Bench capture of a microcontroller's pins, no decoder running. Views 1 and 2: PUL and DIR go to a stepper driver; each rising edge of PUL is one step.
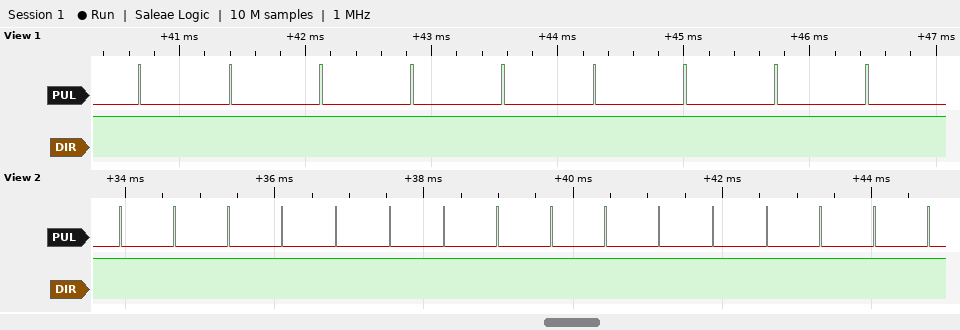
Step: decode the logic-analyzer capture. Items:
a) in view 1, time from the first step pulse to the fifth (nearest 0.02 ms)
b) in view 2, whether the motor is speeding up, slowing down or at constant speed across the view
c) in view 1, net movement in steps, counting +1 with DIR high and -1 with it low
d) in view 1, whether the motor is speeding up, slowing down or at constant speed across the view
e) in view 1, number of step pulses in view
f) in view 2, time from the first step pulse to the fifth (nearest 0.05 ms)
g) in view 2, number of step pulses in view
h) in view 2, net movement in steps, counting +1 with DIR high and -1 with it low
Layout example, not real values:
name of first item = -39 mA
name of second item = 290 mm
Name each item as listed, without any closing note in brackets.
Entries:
in view 1, time from the first step pulse to the fifth = 2.88 ms
in view 2, whether the motor is speeding up, slowing down or at constant speed across the view = constant speed
in view 1, net movement in steps, counting +1 with DIR high and -1 with it low = +9
in view 1, whether the motor is speeding up, slowing down or at constant speed across the view = constant speed
in view 1, number of step pulses in view = 9
in view 2, time from the first step pulse to the fifth = 2.90 ms
in view 2, number of step pulses in view = 16
in view 2, net movement in steps, counting +1 with DIR high and -1 with it low = +16
